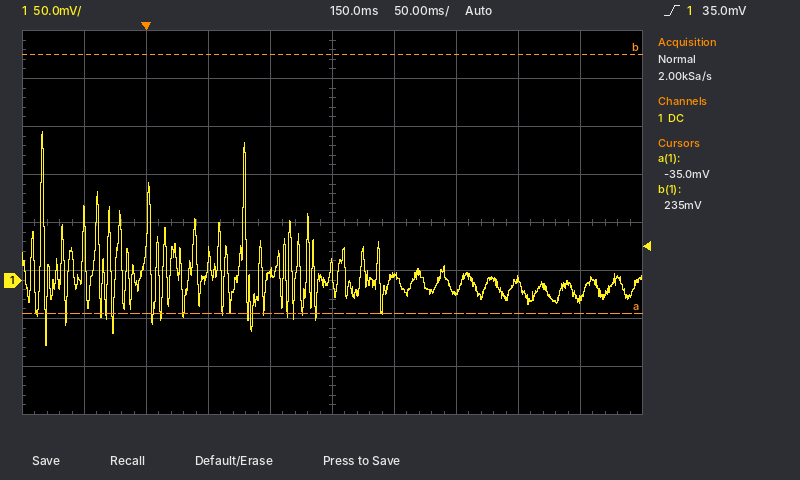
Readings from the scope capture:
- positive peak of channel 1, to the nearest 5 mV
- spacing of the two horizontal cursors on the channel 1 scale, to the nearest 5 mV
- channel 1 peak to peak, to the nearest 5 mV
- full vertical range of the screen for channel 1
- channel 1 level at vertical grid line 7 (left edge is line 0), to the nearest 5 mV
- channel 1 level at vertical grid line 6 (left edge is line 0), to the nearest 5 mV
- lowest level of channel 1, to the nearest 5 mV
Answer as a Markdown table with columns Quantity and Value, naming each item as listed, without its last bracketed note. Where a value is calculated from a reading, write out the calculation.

| Quantity | Value |
|---|---|
| positive peak of channel 1, to the nearest 5 mV | 155 mV |
| spacing of the two horizontal cursors on the channel 1 scale, to the nearest 5 mV | 270 mV |
| channel 1 peak to peak, to the nearest 5 mV | 155 mV − (-70 mV) = 225 mV |
| full vertical range of the screen for channel 1 | 400 mV |
| channel 1 level at vertical grid line 7 (left edge is line 0), to the nearest 5 mV | -15 mV |
| channel 1 level at vertical grid line 6 (left edge is line 0), to the nearest 5 mV | 5 mV |
| lowest level of channel 1, to the nearest 5 mV | -70 mV |
